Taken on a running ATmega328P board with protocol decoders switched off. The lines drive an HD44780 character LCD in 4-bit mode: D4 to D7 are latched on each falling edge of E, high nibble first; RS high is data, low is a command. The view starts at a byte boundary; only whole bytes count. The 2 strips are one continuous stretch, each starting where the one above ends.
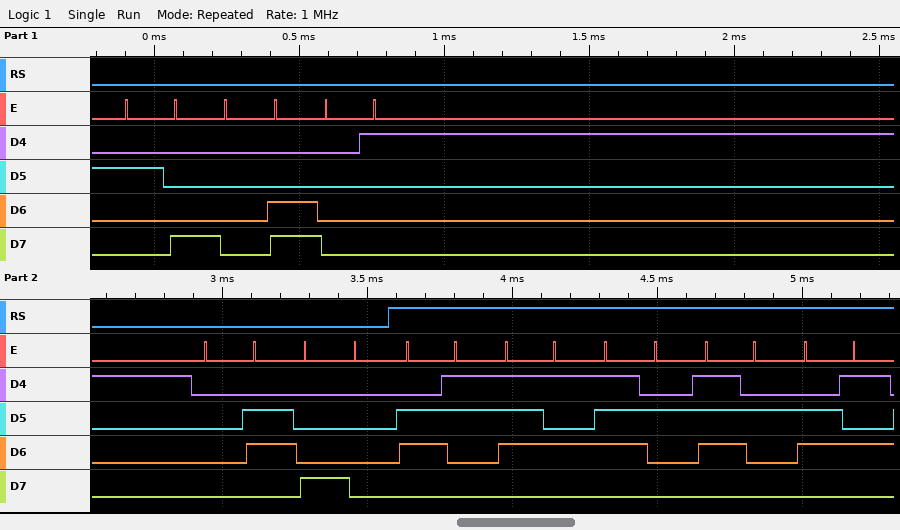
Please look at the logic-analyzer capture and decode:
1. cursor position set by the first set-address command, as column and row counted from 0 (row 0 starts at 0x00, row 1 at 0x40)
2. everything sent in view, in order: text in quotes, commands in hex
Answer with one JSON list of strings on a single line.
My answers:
["column 0, row 0", "0x28 0x0C 0x01 0x06 0x80 \"curre\""]
